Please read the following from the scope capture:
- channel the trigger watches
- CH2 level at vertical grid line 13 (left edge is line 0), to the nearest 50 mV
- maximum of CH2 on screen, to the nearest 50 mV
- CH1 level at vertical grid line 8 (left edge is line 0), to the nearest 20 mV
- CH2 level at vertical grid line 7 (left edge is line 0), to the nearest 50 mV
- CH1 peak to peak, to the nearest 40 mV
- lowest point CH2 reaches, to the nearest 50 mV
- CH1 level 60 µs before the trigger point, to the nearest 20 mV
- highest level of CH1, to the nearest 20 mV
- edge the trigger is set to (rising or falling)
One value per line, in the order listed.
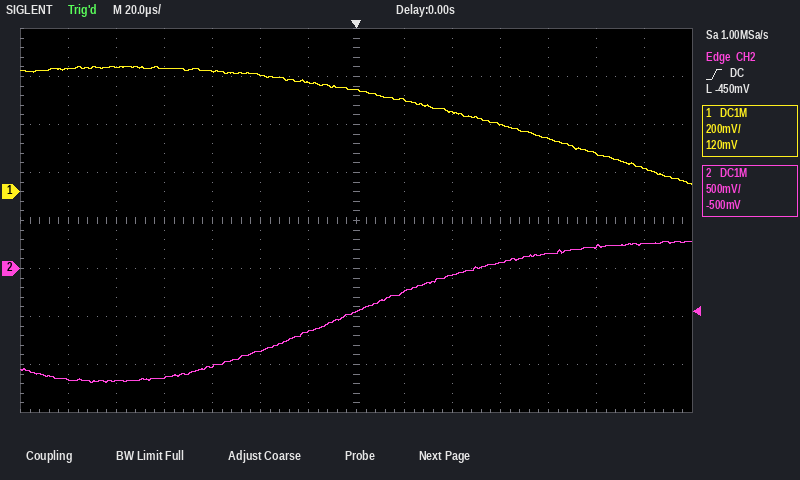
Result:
CH2
250 mV
300 mV
380 mV
-450 mV
480 mV
-1.20 V
500 mV
520 mV
rising
